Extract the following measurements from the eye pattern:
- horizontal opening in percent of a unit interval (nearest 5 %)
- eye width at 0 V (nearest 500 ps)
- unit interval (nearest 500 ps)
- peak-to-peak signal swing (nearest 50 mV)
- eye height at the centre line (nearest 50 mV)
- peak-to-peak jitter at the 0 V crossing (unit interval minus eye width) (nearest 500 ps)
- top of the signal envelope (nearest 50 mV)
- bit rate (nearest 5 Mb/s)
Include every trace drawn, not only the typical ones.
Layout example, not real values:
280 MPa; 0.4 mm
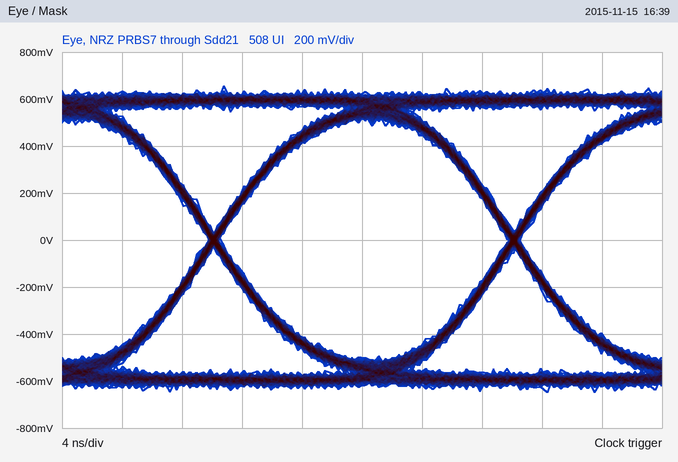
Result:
95 %; 19.0 ns; 20.0 ns; 1.30 V; 1.00 V; 1.0 ns; 650 mV; 50 Mb/s
